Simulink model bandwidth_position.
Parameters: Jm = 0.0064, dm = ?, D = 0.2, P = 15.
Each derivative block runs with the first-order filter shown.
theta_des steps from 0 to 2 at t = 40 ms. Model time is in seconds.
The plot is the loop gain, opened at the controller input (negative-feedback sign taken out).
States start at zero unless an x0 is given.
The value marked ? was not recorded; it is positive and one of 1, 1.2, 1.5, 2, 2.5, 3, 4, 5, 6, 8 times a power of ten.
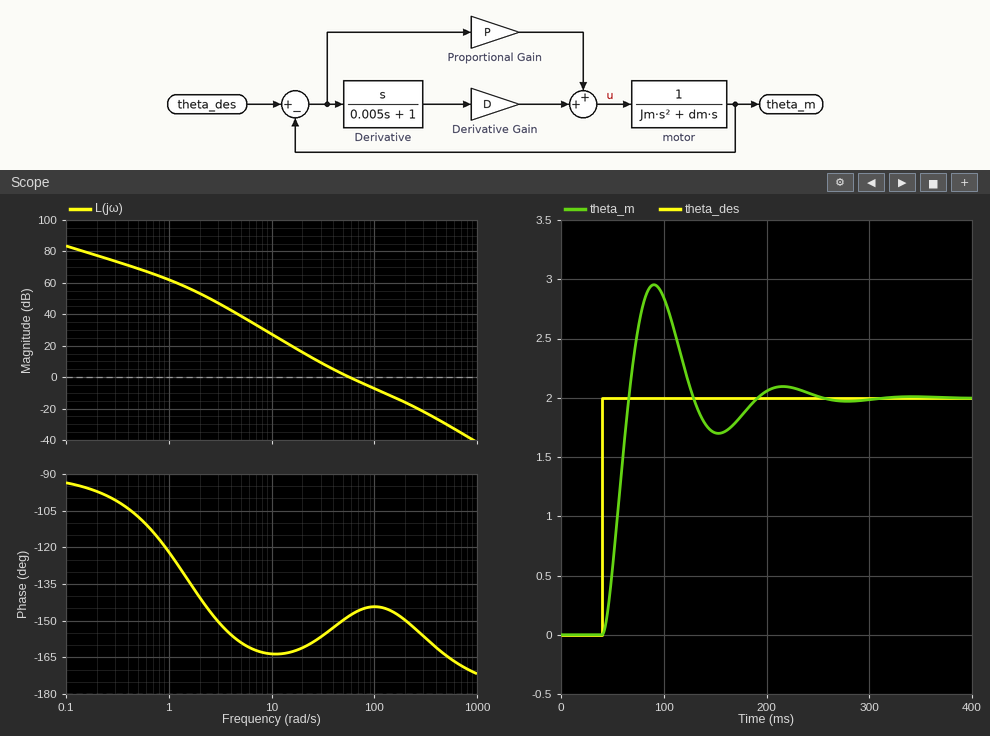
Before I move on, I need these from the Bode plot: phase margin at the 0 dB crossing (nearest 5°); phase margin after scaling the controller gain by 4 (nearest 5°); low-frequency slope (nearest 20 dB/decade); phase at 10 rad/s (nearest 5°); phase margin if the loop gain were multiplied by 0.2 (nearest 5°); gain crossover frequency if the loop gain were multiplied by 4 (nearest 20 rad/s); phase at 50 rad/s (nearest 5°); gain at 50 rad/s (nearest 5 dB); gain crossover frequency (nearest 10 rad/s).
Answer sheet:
30°
35°
-20 dB/decade
-165°
20°
140 rad/s
-150°
0 dB
60 rad/s
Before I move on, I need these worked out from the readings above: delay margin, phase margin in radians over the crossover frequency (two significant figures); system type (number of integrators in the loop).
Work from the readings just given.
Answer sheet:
0.0087 s
1
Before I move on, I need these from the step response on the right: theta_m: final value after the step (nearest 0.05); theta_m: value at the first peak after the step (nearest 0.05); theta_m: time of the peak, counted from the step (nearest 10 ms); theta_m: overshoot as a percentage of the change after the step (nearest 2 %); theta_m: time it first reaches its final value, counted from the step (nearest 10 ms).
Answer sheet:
2.00
2.95
50 ms
48 %
30 ms
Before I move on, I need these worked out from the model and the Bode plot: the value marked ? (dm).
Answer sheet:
0.01
